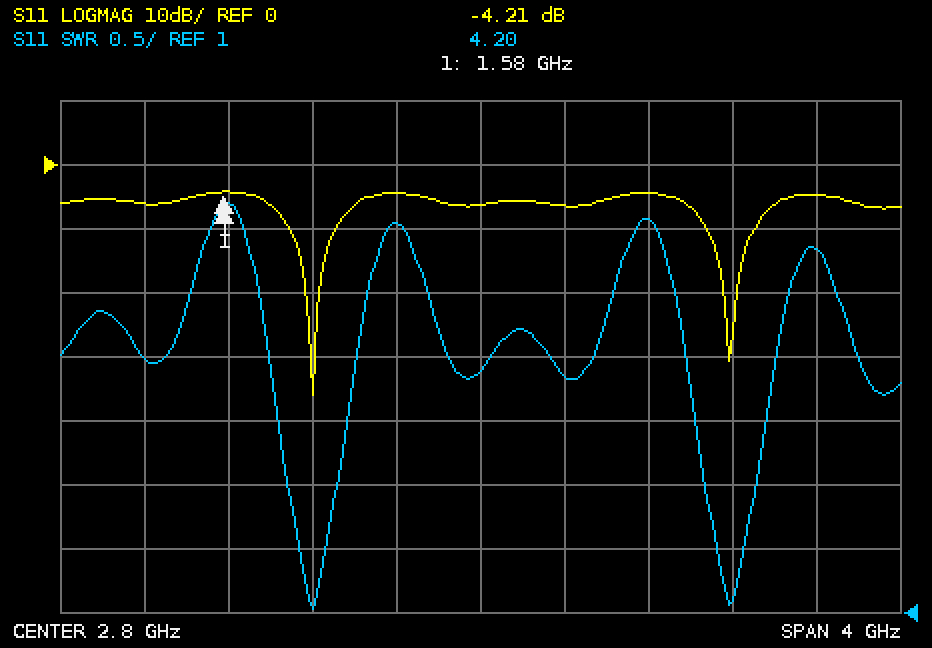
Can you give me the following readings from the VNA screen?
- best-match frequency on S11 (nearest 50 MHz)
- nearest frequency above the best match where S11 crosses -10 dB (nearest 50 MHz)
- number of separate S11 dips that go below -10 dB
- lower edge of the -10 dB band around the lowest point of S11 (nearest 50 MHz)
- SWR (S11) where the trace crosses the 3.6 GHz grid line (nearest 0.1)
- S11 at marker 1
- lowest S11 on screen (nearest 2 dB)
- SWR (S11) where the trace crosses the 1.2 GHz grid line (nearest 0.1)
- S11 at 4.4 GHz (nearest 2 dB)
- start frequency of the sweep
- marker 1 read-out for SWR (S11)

2.00 GHz
2.10 GHz
2
1.90 GHz
4.1
-4.21 dB
-36 dB
3.0
-4 dB
800 MHz
4.20
